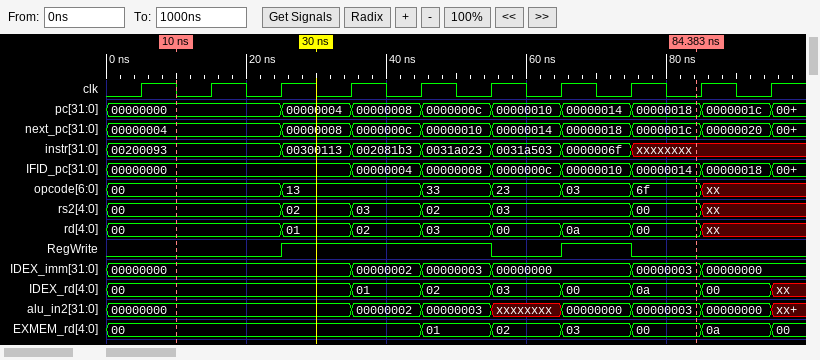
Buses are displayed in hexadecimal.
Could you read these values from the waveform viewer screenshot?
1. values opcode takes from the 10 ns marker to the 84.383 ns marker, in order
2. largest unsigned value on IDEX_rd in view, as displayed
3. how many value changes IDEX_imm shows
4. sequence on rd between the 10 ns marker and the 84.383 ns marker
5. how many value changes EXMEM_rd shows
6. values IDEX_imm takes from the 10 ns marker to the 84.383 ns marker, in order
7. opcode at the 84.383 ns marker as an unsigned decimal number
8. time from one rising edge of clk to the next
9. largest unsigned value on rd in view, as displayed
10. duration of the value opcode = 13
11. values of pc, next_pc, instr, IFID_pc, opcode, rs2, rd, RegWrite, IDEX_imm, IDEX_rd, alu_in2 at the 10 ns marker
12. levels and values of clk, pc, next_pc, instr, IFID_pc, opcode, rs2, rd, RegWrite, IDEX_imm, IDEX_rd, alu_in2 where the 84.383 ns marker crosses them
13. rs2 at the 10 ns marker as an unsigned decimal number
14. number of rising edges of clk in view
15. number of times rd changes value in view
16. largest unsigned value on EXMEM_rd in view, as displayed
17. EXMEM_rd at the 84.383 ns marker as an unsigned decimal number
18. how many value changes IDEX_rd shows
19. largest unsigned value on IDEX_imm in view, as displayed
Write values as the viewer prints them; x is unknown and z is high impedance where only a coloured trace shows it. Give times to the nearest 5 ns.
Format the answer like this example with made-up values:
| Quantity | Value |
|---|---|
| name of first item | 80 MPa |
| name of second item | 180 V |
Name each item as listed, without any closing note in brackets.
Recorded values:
| Quantity | Value |
|---|---|
| values opcode takes from the 10 ns marker to the 84.383 ns marker, in order | 00, 13, 33, 23, 03, 6f |
| largest unsigned value on IDEX_rd in view, as displayed | 0a |
| how many value changes IDEX_imm shows | 5 |
| sequence on rd between the 10 ns marker and the 84.383 ns marker | 00, 01, 02, 03, 00, 0a, 00 |
| how many value changes EXMEM_rd shows | 6 |
| values IDEX_imm takes from the 10 ns marker to the 84.383 ns marker, in order | 00000000, 00000002, 00000003, 00000000, 00000003 |
| opcode at the 84.383 ns marker as an unsigned decimal number | 111 |
| time from one rising edge of clk to the next | 10 ns |
| largest unsigned value on rd in view, as displayed | 0a |
| duration of the value opcode = 13 | 20 ns |
| values of pc, next_pc, instr, IFID_pc, opcode, rs2, rd, RegWrite, IDEX_imm, IDEX_rd, alu_in2 at the 10 ns marker | pc=00000000, next_pc=00000004, instr=00200093, IFID_pc=00000000, opcode=00, rs2=00, rd=00, RegWrite=0, IDEX_imm=00000000, IDEX_rd=00, alu_in2=00000000 |
| levels and values of clk, pc, next_pc, instr, IFID_pc, opcode, rs2, rd, RegWrite, IDEX_imm, IDEX_rd, alu_in2 where the 84.383 ns marker crosses them | clk=0, pc=00000018, next_pc=0000001c, instr=xxxxxxxx, IFID_pc=00000014, opcode=6f, rs2=00, rd=00, RegWrite=0, IDEX_imm=00000003, IDEX_rd=0a, alu_in2=00000003 |
| rs2 at the 10 ns marker as an unsigned decimal number | 0 |
| number of rising edges of clk in view | 10 |
| number of times rd changes value in view | 7 |
| largest unsigned value on EXMEM_rd in view, as displayed | 0a |
| EXMEM_rd at the 84.383 ns marker as an unsigned decimal number | 0 |
| how many value changes IDEX_rd shows | 7 |
| largest unsigned value on IDEX_imm in view, as displayed | 00000003 |
